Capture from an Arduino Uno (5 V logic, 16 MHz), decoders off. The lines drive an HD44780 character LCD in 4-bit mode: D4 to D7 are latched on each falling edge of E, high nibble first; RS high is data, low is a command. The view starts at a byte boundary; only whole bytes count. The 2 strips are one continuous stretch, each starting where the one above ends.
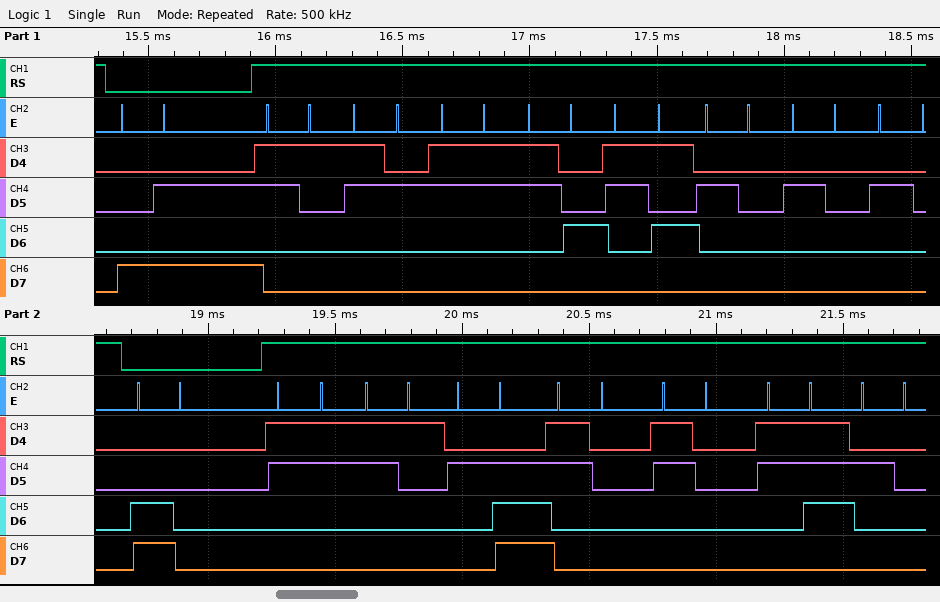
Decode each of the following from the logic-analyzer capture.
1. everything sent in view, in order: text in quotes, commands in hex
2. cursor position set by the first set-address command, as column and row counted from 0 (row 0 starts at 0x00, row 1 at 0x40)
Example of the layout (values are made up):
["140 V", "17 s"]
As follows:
["0x8A \"12345   \" 0xC0 \"31.007 \"", "column 10, row 0"]
